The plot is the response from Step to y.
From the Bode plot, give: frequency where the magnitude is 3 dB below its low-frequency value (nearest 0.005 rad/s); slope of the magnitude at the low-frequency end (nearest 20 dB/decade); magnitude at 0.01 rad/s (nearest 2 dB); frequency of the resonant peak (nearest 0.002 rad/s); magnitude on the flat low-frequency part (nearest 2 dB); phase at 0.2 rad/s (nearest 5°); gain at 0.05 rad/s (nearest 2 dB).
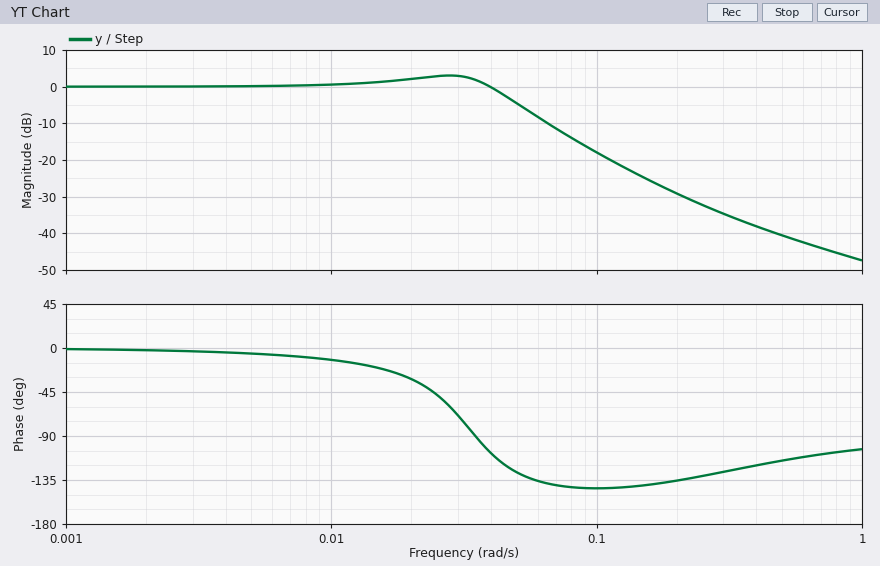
0.045 rad/s
0 dB/decade
0 dB
0.028 rad/s
0 dB
-135°
-4 dB
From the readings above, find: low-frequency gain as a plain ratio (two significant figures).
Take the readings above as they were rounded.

1.0
